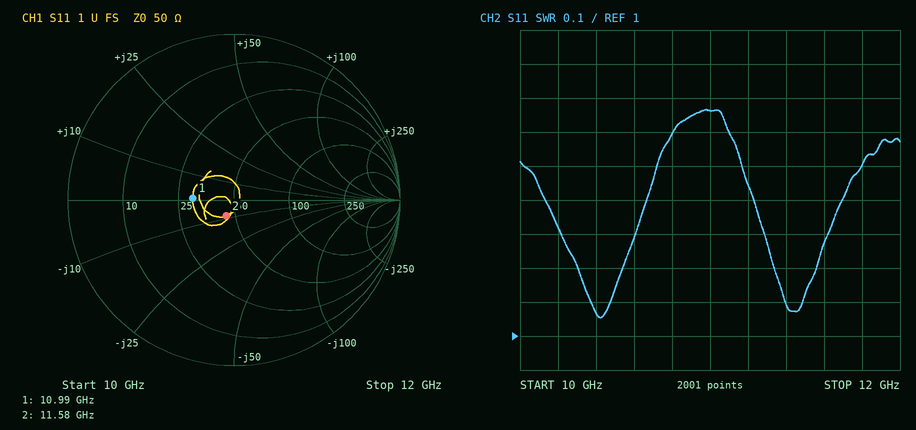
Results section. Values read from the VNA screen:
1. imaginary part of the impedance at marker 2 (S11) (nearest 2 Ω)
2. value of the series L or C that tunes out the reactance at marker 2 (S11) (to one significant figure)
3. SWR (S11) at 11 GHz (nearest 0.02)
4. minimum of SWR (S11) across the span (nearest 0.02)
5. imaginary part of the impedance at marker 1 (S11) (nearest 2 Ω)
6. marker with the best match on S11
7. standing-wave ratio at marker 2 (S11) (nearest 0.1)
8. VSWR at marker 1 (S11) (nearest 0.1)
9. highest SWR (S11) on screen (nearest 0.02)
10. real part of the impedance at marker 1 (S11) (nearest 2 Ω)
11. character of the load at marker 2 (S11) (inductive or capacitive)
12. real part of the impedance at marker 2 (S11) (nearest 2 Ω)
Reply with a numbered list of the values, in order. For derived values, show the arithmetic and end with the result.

1. -8 Ω
2. L = 8 Ω/(2π × 11.58 GHz) ≈ 110 pH, so 100 pH to one significant figure
3. 1.66
4. 1.06
5. 0 Ω
6. marker 2
7. 1.2
8. 1.7
9. 1.66
10. 30 Ω
11. capacitive
12. 44 Ω
